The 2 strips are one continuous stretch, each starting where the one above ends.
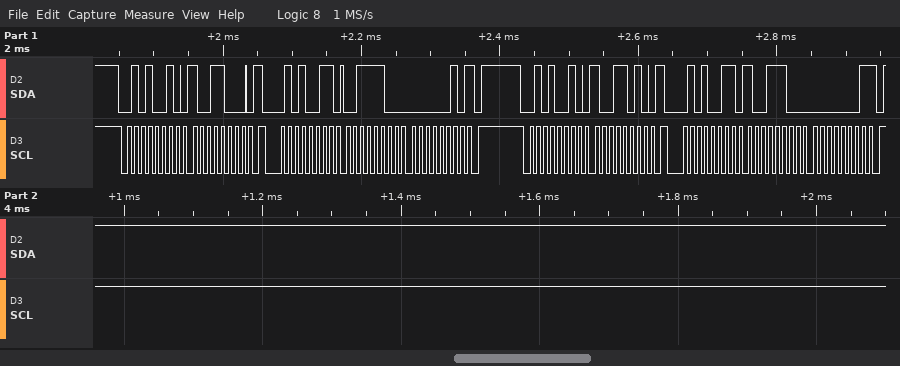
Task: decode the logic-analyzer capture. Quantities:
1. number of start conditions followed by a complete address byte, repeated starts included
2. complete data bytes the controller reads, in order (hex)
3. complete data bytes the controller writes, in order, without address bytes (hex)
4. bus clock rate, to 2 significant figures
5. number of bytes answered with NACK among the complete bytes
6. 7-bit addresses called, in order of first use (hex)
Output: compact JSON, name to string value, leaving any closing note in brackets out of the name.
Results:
{"number of start conditions followed by a complete address byte, repeated starts included": "4", "complete data bytes the controller reads, in order": "3C 02 9C 01", "complete data bytes the controller writes, in order, without address bytes": "98 9A", "bus clock rate, to 2 significant figures": "100 kHz", "number of bytes answered with NACK among the complete bytes": "2", "7-bit addresses called, in order of first use": "0x29"}
